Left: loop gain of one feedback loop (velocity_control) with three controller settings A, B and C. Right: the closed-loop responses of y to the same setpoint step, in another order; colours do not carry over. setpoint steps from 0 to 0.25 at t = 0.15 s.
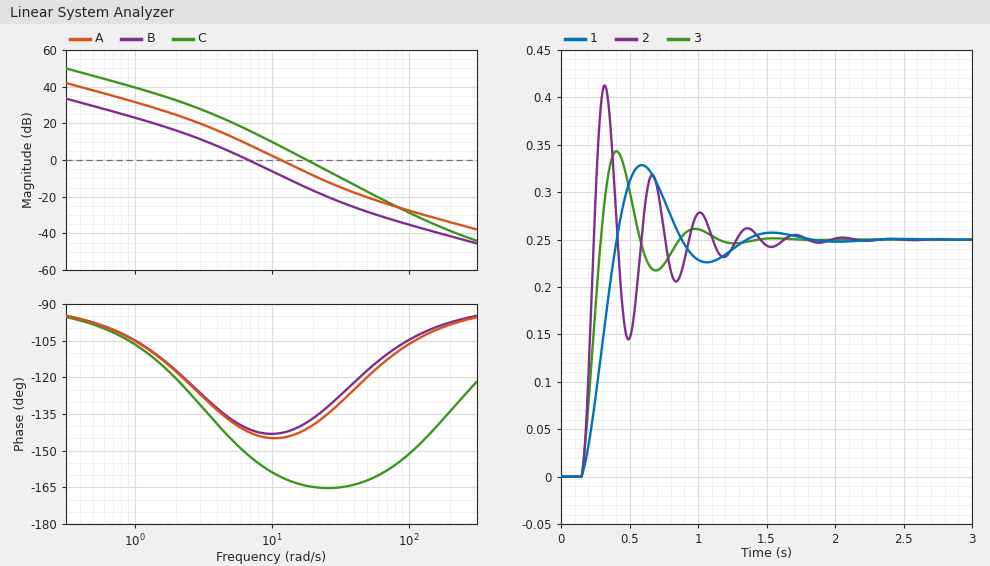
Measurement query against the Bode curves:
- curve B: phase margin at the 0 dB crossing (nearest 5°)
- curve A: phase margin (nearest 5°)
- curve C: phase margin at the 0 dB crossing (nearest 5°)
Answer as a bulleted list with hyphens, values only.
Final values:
- 40°
- 35°
- 15°
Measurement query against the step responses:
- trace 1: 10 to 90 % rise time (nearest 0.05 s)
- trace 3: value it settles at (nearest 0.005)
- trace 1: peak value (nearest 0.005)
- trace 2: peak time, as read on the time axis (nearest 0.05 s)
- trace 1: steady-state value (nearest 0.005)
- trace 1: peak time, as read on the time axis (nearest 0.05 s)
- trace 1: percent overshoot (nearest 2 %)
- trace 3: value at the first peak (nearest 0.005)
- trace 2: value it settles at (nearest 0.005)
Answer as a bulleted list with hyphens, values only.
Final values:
- 0.20 s
- 0.250
- 0.330
- 0.30 s
- 0.250
- 0.60 s
- 32 %
- 0.345
- 0.250
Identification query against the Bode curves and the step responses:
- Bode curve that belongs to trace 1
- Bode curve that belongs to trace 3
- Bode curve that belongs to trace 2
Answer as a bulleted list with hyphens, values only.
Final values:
- B
- A
- C
